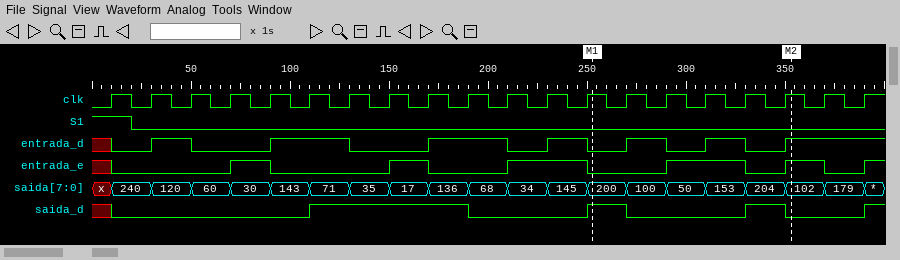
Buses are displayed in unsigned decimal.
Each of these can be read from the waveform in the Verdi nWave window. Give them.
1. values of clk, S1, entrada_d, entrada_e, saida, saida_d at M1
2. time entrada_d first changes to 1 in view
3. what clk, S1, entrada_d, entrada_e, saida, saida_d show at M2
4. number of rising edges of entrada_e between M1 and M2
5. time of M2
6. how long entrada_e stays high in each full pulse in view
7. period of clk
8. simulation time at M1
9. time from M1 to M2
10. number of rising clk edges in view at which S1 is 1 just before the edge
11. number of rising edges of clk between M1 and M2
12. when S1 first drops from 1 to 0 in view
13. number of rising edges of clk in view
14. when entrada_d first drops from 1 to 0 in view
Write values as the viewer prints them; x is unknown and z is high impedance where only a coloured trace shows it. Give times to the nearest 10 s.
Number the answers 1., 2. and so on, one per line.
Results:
1. clk=1, S1=0, entrada_d=0, entrada_e=0, saida=200, saida_d=1
2. 30 s
3. clk=1, S1=0, entrada_d=1, entrada_e=1, saida=102, saida_d=0
4. 2
5. 350 s
6. 20 s, 20 s, 40 s, 40 s, 20 s
7. 20 s
8. 250 s
9. 100 s
10. 1
11. 5
12. 20 s
13. 20
14. 50 s
